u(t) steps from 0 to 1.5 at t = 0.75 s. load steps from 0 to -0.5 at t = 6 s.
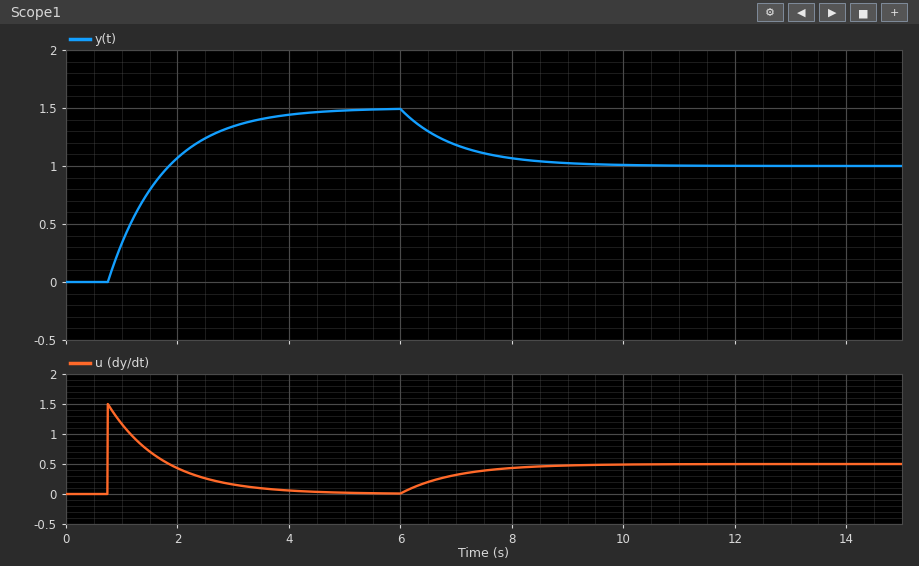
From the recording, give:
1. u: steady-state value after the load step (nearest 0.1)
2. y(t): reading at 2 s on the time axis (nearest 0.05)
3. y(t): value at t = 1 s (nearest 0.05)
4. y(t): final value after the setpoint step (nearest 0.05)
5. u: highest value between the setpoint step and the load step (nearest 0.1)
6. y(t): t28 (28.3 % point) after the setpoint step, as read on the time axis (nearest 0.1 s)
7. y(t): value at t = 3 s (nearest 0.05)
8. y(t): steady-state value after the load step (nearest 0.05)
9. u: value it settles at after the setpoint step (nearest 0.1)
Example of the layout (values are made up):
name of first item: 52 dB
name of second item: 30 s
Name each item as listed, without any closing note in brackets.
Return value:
u: steady-state value after the load step: 0.5
y(t): reading at 2 s on the time axis: 1.05
y(t): value at t = 1 s: 0.35
y(t): final value after the setpoint step: 1.50
u: highest value between the setpoint step and the load step: 1.5
y(t): t28 (28.3 % point) after the setpoint step, as read on the time axis: 1.1 s
y(t): value at t = 3 s: 1.35
y(t): steady-state value after the load step: 1.00
u: value it settles at after the setpoint step: 0.0
